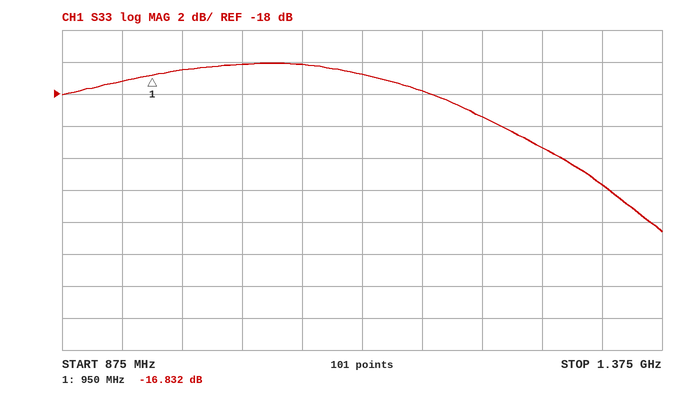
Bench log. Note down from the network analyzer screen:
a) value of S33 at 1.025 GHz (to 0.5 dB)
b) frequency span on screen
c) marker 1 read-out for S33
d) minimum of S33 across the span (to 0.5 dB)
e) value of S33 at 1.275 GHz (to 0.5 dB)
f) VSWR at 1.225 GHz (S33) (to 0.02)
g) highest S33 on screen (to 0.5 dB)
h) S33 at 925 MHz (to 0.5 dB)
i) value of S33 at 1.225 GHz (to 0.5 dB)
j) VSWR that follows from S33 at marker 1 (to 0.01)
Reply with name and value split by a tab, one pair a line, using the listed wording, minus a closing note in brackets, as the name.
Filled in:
value of S33 at 1.025 GHz	-16.0 dB
frequency span on screen	500 MHz
marker 1 read-out for S33	-16.832 dB
minimum of S33 across the span	-26.5 dB
value of S33 at 1.275 GHz	-21.5 dB
VSWR at 1.225 GHz (S33)	1.24
highest S33 on screen	-16.0 dB
S33 at 925 MHz	-17.0 dB
value of S33 at 1.225 GHz	-19.5 dB
VSWR that follows from S33 at marker 1	1.34
